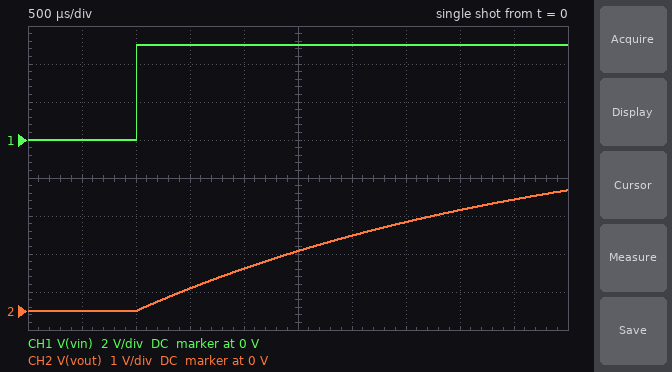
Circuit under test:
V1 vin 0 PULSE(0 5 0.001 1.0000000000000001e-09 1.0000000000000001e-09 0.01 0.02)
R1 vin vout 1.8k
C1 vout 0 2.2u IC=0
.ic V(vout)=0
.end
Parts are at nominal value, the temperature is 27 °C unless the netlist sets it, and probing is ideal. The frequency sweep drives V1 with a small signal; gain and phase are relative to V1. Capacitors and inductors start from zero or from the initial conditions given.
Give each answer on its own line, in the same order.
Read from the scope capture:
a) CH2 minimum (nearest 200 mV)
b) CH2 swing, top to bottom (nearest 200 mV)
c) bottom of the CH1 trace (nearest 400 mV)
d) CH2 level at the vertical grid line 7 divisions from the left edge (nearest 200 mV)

0 V
3.2 V
0 V
2.4 V
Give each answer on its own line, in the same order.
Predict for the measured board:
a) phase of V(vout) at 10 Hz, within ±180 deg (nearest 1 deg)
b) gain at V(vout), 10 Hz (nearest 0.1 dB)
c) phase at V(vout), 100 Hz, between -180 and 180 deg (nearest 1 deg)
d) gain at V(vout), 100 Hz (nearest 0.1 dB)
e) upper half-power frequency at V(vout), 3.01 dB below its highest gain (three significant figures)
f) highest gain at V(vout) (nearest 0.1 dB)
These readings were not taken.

-14 deg
-0.3 dB
-68 deg
-8.6 dB
40.2 Hz
0 dB
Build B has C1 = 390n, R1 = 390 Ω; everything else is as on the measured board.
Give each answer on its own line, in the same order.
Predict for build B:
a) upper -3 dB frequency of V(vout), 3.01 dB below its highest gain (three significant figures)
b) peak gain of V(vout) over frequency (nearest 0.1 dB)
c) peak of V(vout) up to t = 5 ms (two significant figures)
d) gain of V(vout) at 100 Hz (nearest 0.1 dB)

1.05 kHz
0 dB
5.0 V
0 dB
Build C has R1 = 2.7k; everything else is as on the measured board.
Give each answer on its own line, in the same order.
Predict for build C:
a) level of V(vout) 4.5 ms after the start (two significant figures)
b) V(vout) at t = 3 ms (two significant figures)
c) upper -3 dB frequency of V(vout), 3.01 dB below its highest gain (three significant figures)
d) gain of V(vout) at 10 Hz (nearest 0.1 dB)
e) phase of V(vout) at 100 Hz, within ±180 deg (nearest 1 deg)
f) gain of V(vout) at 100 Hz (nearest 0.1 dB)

2.2 V
1.4 V
26.8 Hz
-0.6 dB
-75 deg
-11.7 dB
